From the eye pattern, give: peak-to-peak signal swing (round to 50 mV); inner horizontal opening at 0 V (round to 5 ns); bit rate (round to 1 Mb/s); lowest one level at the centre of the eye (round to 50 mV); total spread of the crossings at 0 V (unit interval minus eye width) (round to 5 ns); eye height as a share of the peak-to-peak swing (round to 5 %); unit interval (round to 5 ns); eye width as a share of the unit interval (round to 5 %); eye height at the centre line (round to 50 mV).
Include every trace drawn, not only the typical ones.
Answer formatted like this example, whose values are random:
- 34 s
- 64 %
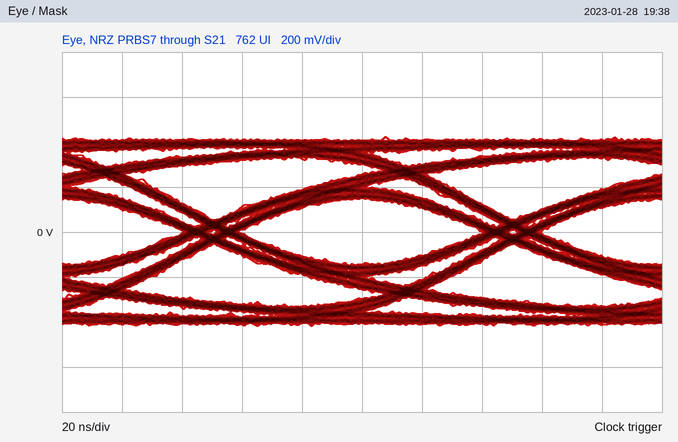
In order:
- 850 mV
- 80 ns
- 10 Mb/s
- 150 mV
- 20 ns
- 35 %
- 100 ns
- 80 %
- 300 mV
